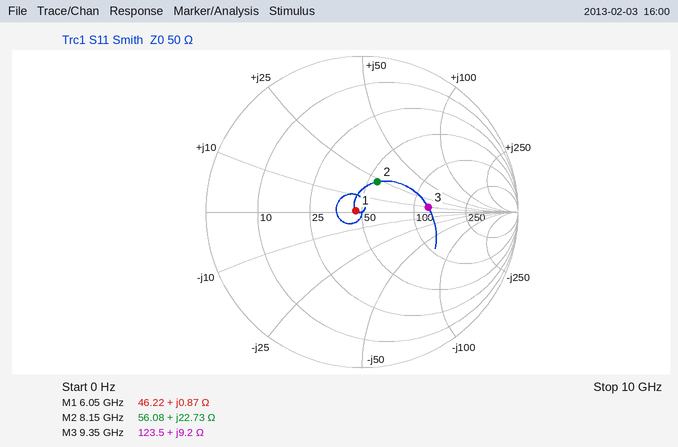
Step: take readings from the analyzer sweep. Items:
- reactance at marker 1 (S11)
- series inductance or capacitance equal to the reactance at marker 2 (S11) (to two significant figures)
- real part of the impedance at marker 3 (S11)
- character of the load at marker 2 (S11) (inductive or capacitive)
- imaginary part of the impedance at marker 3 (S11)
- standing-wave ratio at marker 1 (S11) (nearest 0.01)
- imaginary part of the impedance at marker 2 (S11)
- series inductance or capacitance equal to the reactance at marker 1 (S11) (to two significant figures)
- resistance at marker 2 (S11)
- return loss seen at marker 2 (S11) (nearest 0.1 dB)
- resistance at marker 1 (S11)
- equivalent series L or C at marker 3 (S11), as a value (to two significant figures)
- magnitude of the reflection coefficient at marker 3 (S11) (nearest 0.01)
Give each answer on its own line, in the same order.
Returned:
+0.87 Ω
440 pH
123.5 Ω
inductive
+9.2 Ω
1.08
+22.73 Ω
23 pH
56.08 Ω
13.3 dB
46.22 Ω
160 pH
0.43
